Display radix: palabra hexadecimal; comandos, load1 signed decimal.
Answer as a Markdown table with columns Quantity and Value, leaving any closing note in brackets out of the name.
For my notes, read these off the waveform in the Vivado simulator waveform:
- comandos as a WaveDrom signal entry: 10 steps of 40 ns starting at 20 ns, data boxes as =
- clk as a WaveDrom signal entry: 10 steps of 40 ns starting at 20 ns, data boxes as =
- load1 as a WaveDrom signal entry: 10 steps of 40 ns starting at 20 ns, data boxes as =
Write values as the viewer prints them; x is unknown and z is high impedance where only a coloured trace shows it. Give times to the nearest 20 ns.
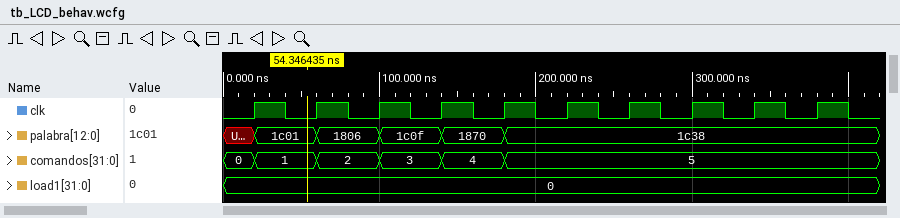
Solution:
| Quantity | Value |
|---|---|
| comandos as a WaveDrom signal entry: 10 steps of 40 ns starting at 20 ns, data boxes as = | {name: 'comandos', wave: '=====.....', data: '1 2 3 4 5'} |
| clk as a WaveDrom signal entry: 10 steps of 40 ns starting at 20 ns, data boxes as = | {name: 'clk', wave: 'p.........'} |
| load1 as a WaveDrom signal entry: 10 steps of 40 ns starting at 20 ns, data boxes as = | {name: 'load1', wave: '=.........', data: '0'} |
